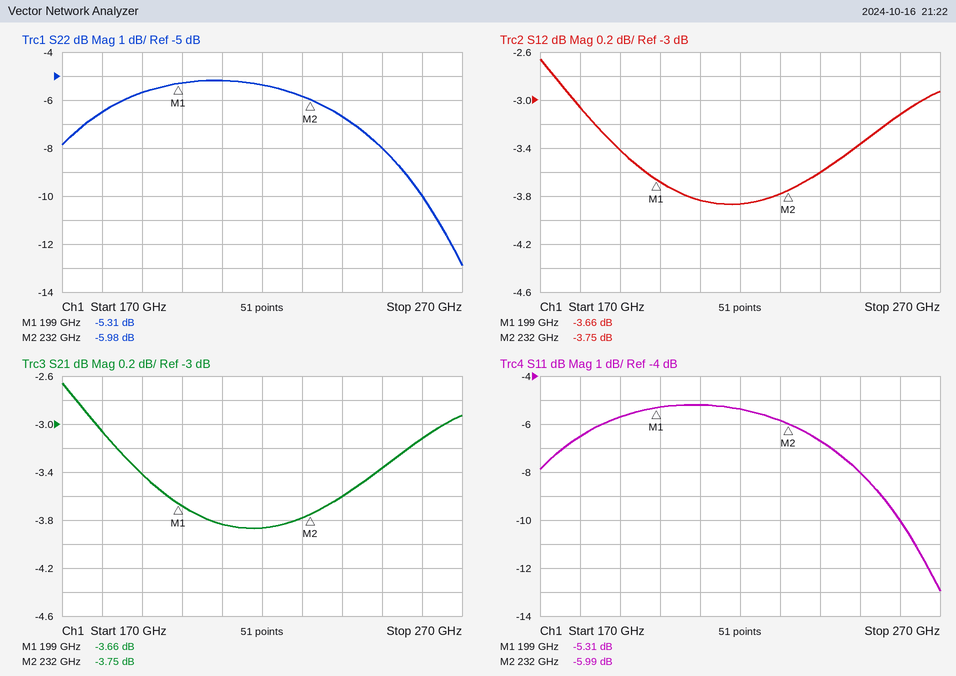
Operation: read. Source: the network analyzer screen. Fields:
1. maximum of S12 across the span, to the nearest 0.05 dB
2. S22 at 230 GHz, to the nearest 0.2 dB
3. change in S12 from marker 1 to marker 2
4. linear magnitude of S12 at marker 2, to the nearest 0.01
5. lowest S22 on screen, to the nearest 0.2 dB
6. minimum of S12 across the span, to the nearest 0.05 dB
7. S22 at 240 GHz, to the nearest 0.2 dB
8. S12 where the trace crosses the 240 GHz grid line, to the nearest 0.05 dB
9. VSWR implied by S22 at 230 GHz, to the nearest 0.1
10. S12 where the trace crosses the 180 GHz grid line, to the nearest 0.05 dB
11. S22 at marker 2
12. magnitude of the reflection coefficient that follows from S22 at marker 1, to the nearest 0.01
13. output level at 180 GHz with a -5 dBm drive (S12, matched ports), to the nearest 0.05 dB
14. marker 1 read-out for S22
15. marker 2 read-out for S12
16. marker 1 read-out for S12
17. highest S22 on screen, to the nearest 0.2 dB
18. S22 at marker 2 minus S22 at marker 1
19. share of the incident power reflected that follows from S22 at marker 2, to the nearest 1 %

-2.65 dB
-5.8 dB
-0.09 dB
0.65
-12.8 dB
-3.85 dB
-6.6 dB
-3.60 dB
3.1
-3.05 dB
-5.98 dB
0.54
-8.05 dBm
-5.31 dB
-3.75 dB
-3.66 dB
-5.2 dB
-0.67 dB
25 %
